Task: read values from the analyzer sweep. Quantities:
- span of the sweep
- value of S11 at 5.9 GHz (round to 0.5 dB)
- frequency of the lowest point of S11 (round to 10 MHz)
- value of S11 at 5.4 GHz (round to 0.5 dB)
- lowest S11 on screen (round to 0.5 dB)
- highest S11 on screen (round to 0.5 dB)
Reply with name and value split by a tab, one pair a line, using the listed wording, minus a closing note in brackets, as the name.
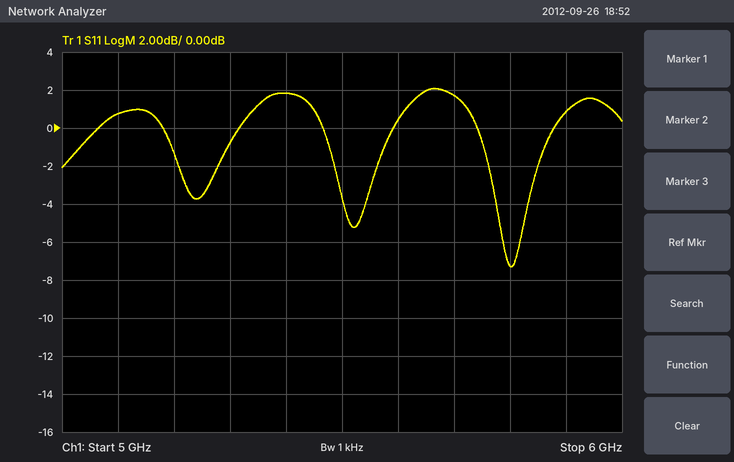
span of the sweep	1 GHz
value of S11 at 5.9 GHz	1.0 dB
frequency of the lowest point of S11	5.80 GHz
value of S11 at 5.4 GHz	2.0 dB
lowest S11 on screen	-7.5 dB
highest S11 on screen	2.0 dB
